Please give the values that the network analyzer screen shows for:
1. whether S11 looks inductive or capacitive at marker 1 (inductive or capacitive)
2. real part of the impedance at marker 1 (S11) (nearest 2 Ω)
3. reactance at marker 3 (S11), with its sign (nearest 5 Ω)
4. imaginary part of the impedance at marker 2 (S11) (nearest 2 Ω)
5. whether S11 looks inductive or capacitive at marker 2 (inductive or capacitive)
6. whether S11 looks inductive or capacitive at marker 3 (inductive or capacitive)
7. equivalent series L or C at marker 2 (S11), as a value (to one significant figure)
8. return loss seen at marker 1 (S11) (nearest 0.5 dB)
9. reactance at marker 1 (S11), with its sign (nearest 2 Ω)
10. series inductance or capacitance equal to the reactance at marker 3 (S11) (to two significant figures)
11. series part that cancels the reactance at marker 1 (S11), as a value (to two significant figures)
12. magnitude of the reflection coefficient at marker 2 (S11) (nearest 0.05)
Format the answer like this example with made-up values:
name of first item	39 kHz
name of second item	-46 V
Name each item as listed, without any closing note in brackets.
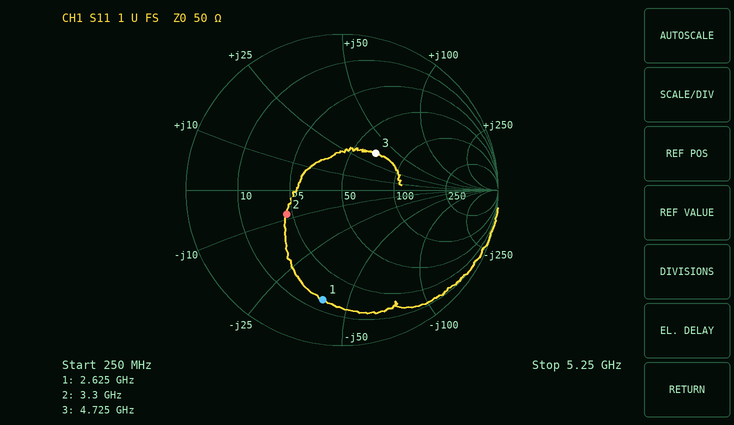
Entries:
whether S11 looks inductive or capacitive at marker 1	capacitive
real part of the impedance at marker 1 (S11)	14 Ω
reactance at marker 3 (S11), with its sign	+35 Ω
imaginary part of the impedance at marker 2 (S11)	-8 Ω
whether S11 looks inductive or capacitive at marker 2	capacitive
whether S11 looks inductive or capacitive at marker 3	inductive
equivalent series L or C at marker 2 (S11), as a value	6 pF
return loss seen at marker 1 (S11)	3.0 dB
reactance at marker 1 (S11), with its sign	-40 Ω
series inductance or capacitance equal to the reactance at marker 3 (S11)	1.2 nH
series part that cancels the reactance at marker 1 (S11), as a value	2.4 nH
magnitude of the reflection coefficient at marker 2 (S11)	0.40
